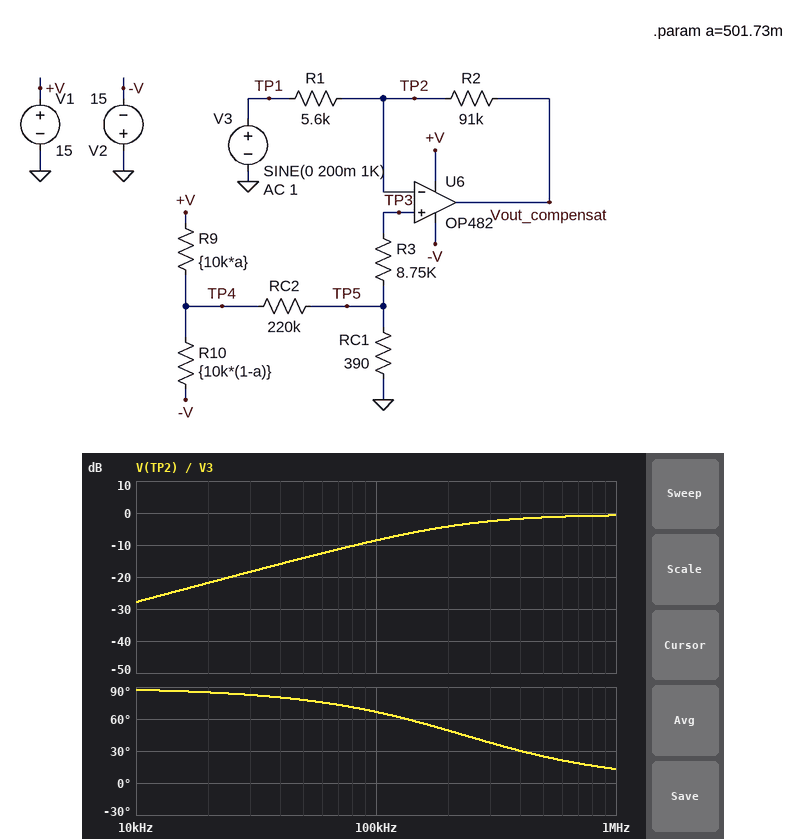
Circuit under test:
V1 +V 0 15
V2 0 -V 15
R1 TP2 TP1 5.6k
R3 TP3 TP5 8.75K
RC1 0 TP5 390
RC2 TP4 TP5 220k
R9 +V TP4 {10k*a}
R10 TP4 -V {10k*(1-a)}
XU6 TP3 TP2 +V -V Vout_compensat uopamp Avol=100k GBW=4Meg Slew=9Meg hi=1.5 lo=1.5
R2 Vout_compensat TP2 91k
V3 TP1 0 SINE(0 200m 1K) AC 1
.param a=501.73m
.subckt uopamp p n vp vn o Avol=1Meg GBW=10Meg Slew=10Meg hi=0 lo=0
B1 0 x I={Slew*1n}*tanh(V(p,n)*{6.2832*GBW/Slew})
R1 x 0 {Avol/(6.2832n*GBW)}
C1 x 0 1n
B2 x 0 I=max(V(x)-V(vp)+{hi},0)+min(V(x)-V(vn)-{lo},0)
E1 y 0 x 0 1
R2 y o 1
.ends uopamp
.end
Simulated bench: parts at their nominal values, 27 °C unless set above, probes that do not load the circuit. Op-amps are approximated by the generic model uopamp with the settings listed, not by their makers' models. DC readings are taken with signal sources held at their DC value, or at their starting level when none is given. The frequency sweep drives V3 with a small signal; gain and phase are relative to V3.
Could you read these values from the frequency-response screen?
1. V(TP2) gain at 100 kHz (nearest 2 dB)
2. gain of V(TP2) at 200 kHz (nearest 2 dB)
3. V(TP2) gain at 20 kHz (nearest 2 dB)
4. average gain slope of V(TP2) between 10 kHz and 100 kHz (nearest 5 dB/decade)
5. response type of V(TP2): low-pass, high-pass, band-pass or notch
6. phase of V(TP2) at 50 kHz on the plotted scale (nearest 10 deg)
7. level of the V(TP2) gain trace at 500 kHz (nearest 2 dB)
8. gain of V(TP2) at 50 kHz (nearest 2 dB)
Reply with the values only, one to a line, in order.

-8 dB
-4 dB
-22 dB
20 dB/decade
high-pass
80 deg
-2 dB
-14 dB
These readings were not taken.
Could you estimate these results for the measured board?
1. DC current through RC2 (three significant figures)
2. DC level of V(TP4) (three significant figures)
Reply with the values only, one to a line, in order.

233 nA
-51.3 mV
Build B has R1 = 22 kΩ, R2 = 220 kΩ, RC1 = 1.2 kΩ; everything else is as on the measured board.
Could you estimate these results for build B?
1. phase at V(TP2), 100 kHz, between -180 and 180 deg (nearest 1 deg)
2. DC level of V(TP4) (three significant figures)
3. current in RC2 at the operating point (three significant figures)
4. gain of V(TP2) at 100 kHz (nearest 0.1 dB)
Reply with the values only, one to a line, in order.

75 deg
-51.3 mV
232 nA
-12.4 dB
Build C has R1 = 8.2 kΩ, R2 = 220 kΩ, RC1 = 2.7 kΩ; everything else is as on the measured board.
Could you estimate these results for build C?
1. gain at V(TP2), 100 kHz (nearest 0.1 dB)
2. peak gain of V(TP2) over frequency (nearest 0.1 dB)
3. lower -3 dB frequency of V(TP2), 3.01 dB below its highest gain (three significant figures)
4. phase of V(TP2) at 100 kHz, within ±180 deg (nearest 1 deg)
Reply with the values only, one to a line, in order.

-5.2 dB
-0.3 dB
144 kHz
55 deg
